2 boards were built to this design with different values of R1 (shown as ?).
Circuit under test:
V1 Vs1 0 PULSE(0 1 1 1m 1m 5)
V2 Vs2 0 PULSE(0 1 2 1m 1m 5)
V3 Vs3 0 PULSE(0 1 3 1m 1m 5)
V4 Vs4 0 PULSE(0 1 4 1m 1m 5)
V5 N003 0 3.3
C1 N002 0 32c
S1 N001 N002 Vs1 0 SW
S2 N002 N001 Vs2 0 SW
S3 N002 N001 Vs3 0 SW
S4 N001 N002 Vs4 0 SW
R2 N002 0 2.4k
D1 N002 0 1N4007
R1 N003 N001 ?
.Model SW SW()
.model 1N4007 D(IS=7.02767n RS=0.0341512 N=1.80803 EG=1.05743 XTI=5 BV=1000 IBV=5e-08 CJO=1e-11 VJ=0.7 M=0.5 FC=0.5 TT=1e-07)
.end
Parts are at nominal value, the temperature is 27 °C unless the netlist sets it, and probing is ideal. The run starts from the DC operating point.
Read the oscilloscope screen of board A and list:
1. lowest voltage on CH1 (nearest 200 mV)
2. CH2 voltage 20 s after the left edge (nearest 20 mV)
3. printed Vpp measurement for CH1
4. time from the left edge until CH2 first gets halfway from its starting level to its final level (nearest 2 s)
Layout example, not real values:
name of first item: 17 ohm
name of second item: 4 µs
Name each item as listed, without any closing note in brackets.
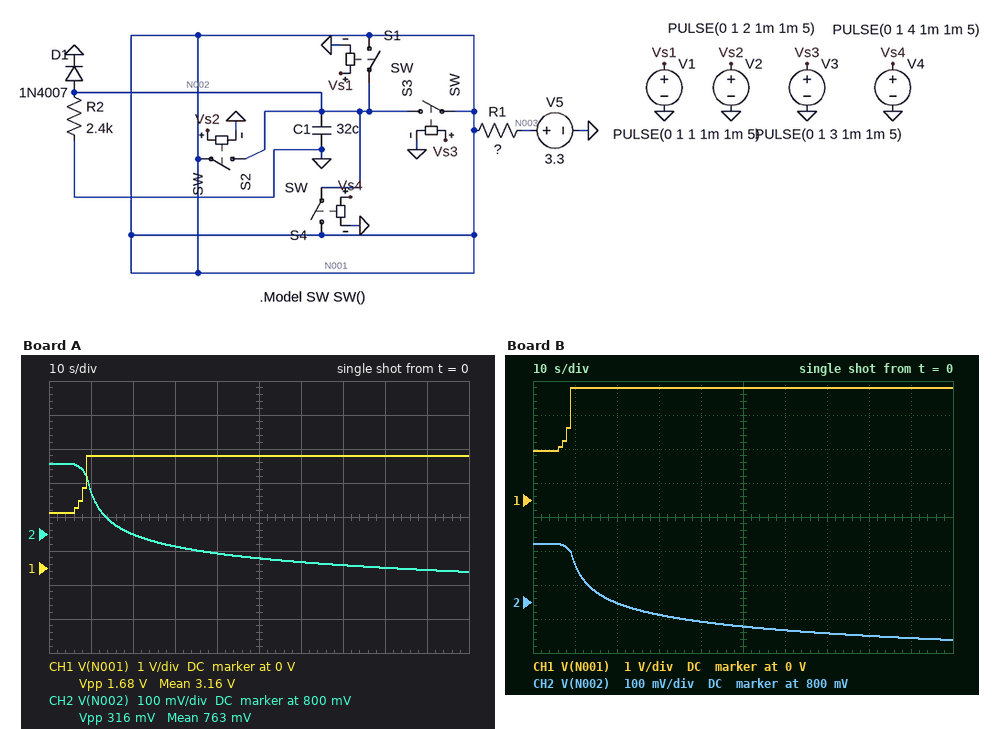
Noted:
lowest voltage on CH1: 1.6 V
CH2 voltage 20 s after the left edge: 800 mV
printed Vpp measurement for CH1: 1.68 V
time from the left edge until CH2 first gets halfway from its starting level to its final level: 14 s
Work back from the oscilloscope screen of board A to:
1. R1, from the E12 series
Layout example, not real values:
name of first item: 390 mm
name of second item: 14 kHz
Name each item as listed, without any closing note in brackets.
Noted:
R1, from the E12 series: 0.68 Ω
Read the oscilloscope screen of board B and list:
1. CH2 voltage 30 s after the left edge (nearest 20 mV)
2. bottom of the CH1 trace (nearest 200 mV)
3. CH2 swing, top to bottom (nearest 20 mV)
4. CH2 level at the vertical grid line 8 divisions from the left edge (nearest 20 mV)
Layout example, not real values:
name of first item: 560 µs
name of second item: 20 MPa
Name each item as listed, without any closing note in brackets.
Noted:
CH2 voltage 30 s after the left edge: 760 mV
bottom of the CH1 trace: 1.4 V
CH2 swing, top to bottom: 280 mV
CH2 level at the vertical grid line 8 divisions from the left edge: 700 mV
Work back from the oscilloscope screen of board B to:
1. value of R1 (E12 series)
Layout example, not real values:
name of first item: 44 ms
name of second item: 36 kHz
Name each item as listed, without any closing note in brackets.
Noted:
value of R1: 1 Ω
